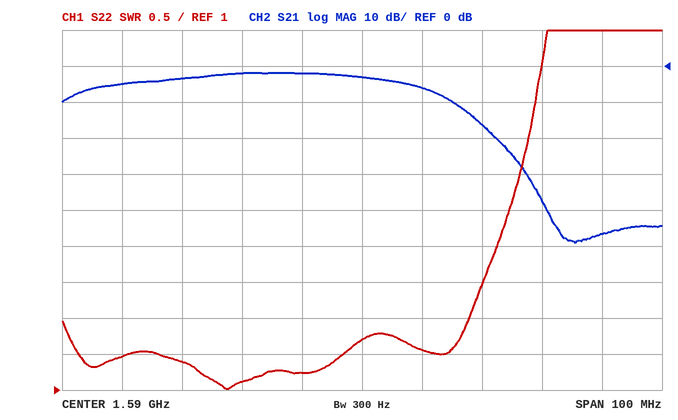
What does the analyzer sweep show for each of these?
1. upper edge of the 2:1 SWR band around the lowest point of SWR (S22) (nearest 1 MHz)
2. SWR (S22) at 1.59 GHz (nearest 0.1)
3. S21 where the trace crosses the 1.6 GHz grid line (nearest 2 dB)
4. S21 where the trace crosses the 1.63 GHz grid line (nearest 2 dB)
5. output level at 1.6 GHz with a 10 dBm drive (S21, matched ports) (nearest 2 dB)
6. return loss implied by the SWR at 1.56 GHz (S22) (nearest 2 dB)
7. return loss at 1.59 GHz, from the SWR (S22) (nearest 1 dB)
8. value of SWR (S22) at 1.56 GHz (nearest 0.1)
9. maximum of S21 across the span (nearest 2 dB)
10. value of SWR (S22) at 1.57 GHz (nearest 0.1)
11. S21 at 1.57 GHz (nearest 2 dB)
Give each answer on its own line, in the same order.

1.608 GHz
1.7
-6 dB
-46 dB
4 dBm
16 dB
12 dB
1.4
-2 dB
1.1
-2 dB
